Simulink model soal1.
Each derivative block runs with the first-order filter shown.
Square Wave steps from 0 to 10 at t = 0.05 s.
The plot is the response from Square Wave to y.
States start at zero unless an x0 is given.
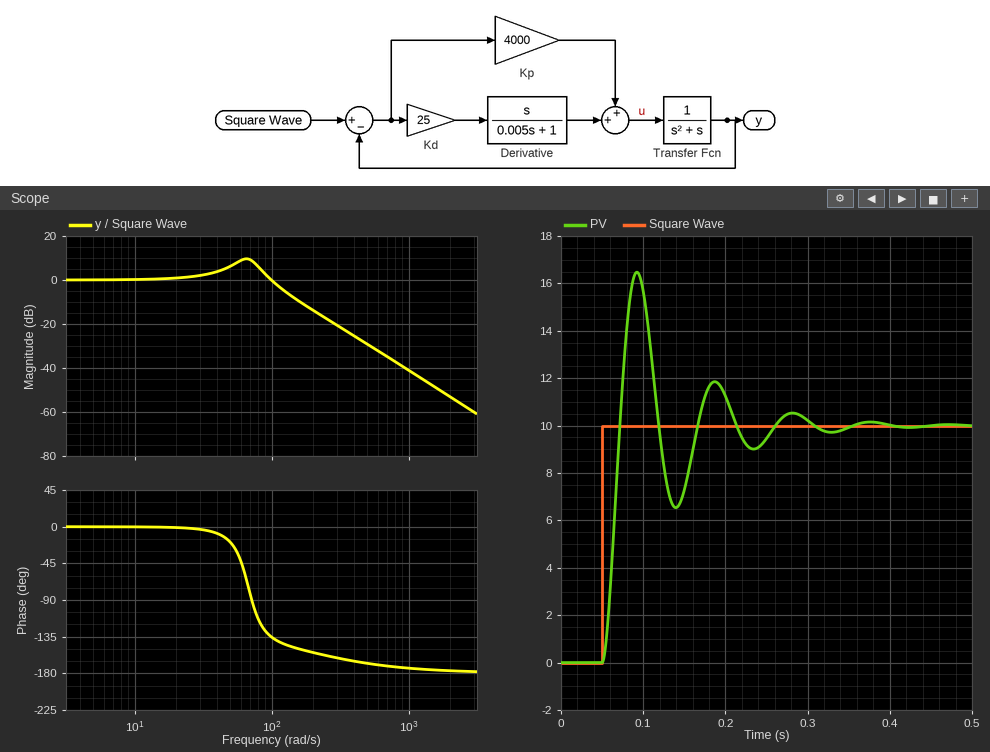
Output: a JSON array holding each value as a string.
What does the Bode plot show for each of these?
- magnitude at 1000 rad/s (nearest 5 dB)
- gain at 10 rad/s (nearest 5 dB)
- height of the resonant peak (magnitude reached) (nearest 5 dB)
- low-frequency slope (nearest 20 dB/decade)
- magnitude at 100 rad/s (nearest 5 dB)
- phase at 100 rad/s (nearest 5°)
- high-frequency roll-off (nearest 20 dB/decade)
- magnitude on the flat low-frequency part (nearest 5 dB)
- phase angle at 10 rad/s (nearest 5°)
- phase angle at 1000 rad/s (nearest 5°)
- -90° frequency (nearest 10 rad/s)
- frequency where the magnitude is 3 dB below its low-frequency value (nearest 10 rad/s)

["-40 dB", "0 dB", "10 dB", "0 dB/decade", "0 dB", "-135°", "-40 dB/decade", "0 dB", "0°", "-175°", "70 rad/s", "110 rad/s"]
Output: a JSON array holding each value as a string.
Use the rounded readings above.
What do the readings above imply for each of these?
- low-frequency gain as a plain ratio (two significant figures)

["1.0"]
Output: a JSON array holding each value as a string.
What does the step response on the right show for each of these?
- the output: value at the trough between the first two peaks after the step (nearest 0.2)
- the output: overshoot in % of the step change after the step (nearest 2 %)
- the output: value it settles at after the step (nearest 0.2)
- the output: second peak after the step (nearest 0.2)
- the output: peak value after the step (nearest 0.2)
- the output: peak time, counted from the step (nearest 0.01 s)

["6.6", "64 %", "10.0", "11.8", "16.4", "0.04 s"]
